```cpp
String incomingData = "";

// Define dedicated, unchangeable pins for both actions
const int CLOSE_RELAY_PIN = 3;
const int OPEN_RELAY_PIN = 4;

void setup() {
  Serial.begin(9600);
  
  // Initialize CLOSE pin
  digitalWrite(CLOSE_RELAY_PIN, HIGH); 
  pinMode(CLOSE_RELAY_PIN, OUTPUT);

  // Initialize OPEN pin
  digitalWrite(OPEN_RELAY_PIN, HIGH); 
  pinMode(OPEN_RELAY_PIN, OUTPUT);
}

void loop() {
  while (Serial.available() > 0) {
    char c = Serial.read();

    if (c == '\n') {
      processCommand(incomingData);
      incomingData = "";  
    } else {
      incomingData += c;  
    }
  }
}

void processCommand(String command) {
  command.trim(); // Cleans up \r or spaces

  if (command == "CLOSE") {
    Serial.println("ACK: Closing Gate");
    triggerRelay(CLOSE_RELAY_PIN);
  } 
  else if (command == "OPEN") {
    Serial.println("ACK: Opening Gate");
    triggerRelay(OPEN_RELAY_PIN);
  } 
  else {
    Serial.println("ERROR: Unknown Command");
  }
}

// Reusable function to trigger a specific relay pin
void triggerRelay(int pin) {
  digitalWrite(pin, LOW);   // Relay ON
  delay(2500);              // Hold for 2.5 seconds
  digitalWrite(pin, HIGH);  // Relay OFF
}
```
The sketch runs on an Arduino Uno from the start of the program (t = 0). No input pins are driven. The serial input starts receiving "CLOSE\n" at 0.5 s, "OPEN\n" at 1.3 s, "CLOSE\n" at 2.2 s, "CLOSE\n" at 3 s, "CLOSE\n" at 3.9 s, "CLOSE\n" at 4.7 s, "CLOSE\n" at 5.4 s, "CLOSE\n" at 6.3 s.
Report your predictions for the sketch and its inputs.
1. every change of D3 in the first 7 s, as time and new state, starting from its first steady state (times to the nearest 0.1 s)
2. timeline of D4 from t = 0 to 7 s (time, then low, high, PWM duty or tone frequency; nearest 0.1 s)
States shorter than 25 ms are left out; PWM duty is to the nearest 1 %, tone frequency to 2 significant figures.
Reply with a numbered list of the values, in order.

1. 0 s high; 0.5 s low; 3 s high; 5.5 s low
2. 0 s high; 3 s low; 5.5 s high
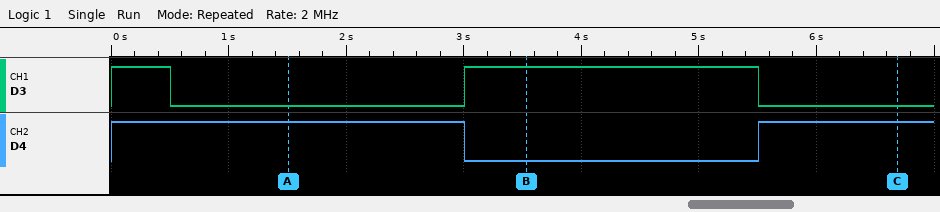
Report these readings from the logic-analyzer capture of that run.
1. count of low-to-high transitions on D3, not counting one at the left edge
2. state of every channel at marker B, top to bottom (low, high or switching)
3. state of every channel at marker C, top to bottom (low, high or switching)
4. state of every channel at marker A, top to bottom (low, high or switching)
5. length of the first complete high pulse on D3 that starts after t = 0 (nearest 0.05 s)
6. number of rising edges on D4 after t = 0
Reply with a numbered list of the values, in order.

1. 1
2. D3 high, D4 low
3. D3 low, D4 high
4. D3 low, D4 high
5. 2.50 s
6. 1
